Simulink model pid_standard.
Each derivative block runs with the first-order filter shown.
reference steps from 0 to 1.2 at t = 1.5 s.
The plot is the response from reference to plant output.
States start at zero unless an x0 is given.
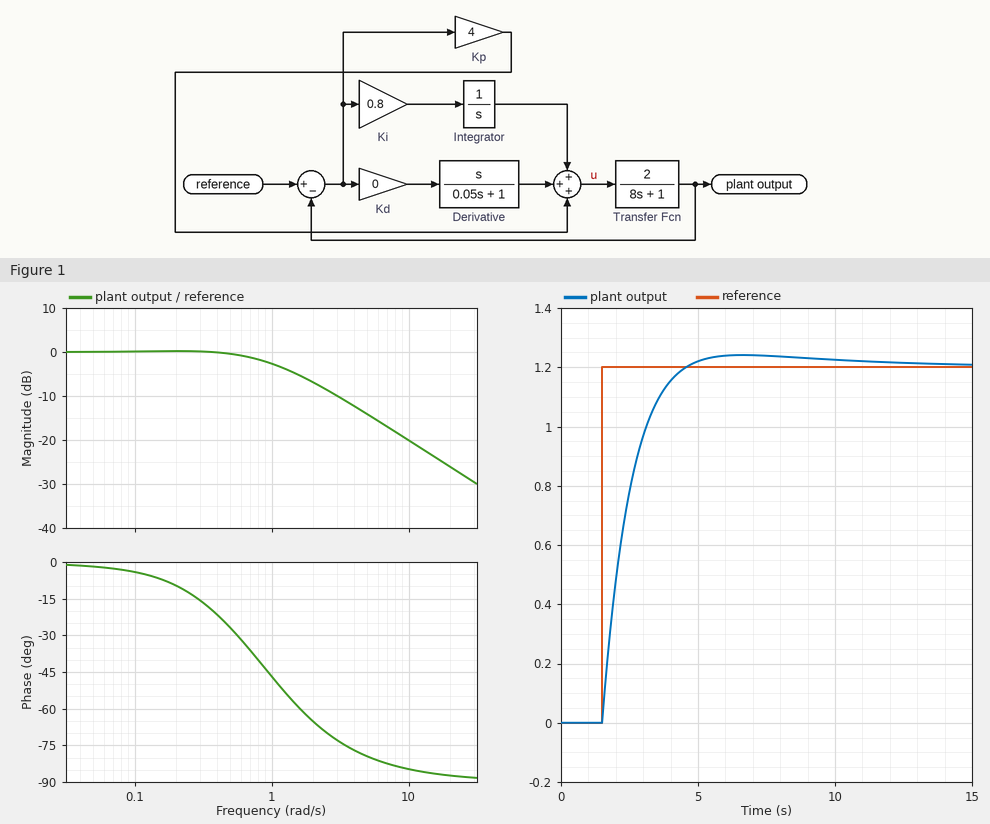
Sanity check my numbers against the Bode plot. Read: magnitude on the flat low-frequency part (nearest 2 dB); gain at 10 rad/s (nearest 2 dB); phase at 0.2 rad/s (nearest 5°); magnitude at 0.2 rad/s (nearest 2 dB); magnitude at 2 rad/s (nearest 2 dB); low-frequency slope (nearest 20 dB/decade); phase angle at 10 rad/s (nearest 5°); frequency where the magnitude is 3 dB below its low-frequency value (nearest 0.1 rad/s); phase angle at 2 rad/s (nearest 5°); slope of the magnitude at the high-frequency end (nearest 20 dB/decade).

0 dB
-20 dB
-10°
0 dB
-6 dB
0 dB/decade
-85°
1.1 rad/s
-65°
-20 dB/decade
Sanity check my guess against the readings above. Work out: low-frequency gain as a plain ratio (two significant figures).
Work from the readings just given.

1.0
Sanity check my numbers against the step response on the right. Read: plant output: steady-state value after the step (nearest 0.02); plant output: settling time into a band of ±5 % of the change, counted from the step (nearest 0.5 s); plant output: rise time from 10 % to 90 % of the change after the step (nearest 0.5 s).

1.20
2.5 s
2.0 s
